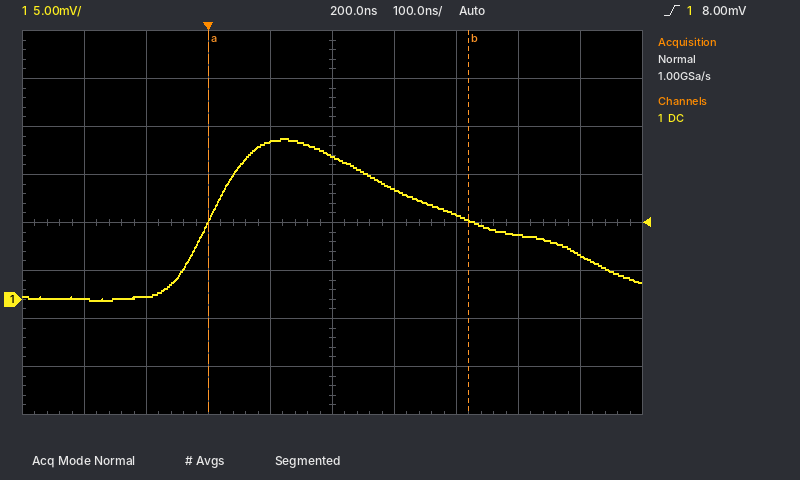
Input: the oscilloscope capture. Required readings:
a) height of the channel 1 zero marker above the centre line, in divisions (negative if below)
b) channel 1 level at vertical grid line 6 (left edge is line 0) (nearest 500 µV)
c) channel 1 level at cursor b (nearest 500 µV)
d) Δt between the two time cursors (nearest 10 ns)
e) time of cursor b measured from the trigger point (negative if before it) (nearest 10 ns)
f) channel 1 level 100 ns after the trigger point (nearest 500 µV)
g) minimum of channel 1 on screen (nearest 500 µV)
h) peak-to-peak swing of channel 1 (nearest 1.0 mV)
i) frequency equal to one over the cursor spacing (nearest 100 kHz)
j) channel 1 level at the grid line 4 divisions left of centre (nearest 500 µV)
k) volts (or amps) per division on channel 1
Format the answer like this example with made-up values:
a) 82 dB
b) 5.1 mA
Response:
a) -1.6 div
b) 11.5 mV
c) 8.0 mV
d) 420 ns
e) +420 ns
f) 16.5 mV
g) 0.0 mV
h) 17.0 mV
i) 2.4 MHz
j) 0.0 mV
k) 5 mV
